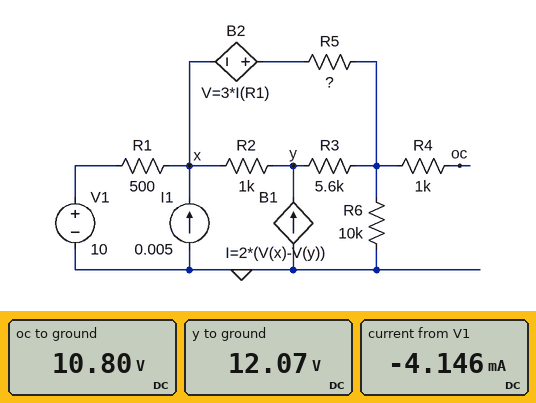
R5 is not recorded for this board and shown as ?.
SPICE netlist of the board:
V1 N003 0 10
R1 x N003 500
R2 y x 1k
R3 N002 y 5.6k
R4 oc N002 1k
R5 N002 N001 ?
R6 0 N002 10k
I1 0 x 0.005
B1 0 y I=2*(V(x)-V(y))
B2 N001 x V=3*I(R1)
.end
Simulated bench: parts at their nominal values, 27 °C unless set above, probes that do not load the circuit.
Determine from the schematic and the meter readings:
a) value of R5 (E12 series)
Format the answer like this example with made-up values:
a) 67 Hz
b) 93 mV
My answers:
a) 1.5 kΩ
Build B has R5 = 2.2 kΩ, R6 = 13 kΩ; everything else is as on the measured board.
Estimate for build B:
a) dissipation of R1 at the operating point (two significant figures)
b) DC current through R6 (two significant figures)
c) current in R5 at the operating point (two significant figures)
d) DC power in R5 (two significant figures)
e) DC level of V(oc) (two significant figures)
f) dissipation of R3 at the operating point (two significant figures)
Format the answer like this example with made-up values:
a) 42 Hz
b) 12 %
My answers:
a) 9.7 mW
b) 840 µA
c) 600 µA
d) 800 µW
e) 11 V
f) 310 µW
